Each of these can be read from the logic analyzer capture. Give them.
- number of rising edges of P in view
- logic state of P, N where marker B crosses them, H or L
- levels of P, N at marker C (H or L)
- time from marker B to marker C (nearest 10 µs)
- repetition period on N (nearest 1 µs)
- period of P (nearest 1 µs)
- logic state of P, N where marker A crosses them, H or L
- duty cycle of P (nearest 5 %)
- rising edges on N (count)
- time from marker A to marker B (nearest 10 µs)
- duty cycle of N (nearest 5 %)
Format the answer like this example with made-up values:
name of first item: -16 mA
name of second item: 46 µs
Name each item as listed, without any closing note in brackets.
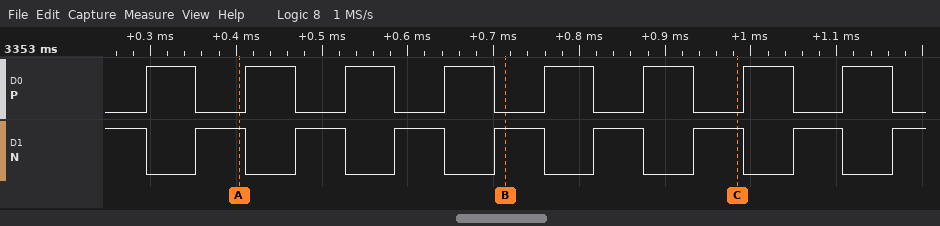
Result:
number of rising edges of P in view: 8
logic state of P, N where marker B crosses them, H or L: P=L, N=H
levels of P, N at marker C: P=L, N=H
time from marker B to marker C: 270 µs
repetition period on N: 116 µs
period of P: 116 µs
logic state of P, N where marker A crosses them, H or L: P=L, N=H
duty cycle of P: 50 %
rising edges on N: 8
time from marker A to marker B: 310 µs
duty cycle of N: 50 %
